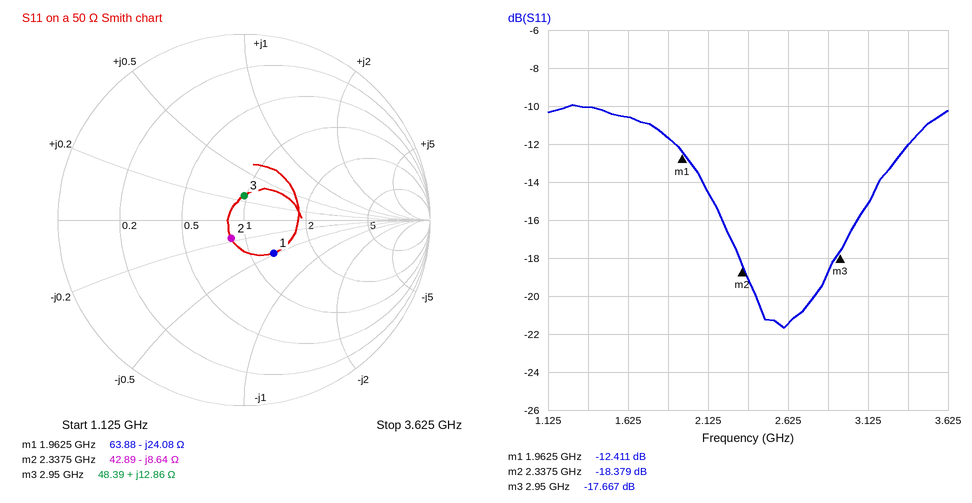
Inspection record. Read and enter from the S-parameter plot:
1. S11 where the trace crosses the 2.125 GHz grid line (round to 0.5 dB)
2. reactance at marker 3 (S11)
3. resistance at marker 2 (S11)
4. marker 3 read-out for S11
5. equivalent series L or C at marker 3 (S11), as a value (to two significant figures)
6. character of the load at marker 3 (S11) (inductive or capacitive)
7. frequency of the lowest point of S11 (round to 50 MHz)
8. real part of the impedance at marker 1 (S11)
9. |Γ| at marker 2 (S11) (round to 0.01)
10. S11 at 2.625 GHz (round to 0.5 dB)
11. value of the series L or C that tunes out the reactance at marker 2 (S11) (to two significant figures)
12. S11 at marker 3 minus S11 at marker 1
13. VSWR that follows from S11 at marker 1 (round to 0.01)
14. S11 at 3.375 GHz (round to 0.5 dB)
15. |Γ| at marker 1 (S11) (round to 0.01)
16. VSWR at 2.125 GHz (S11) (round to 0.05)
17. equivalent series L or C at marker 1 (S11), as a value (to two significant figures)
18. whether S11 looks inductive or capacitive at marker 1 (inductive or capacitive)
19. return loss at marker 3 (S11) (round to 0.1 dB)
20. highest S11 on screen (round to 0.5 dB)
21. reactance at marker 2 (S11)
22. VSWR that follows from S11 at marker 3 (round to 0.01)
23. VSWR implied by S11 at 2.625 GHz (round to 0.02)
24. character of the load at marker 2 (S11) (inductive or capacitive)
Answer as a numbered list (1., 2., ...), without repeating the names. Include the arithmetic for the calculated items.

1. -14.5 dB
2. +12.86 Ω
3. 42.89 Ω
4. -17.667 dB
5. L = 12.86 Ω/(2π × 2.95 GHz) ≈ 694 pH, so 690 pH to two significant figures
6. inductive
7. 2.60 GHz
8. 63.88 Ω
9. 0.12
10. -21.5 dB
11. L = 8.64 Ω/(2π × 2.3375 GHz) ≈ 588 pH, so 590 pH to two significant figures
12. -17.667 − (-12.411) = -5.256 dB
13. (1 + 0.2396)/(1 − 0.2396) ≈ 1.63
14. -12.0 dB
15. 0.24
16. |Γ| = 10^(-14.5/20) = 0.1884; VSWR = (1 + 0.1884)/(1 − 0.1884) ≈ 1.46, so 1.45 to the nearest 0.05
17. C = 1/(2π × 1.9625 GHz × 24.08 Ω) ≈ 3.4 pF
18. capacitive
19. 17.7 dB
20. -10.0 dB
21. -8.64 Ω
22. (1 + 0.1308)/(1 − 0.1308) ≈ 1.30
23. |Γ| = 10^(-21.5/20) = 0.0841; VSWR = (1 + 0.0841)/(1 − 0.0841) ≈ 1.18
24. capacitive
